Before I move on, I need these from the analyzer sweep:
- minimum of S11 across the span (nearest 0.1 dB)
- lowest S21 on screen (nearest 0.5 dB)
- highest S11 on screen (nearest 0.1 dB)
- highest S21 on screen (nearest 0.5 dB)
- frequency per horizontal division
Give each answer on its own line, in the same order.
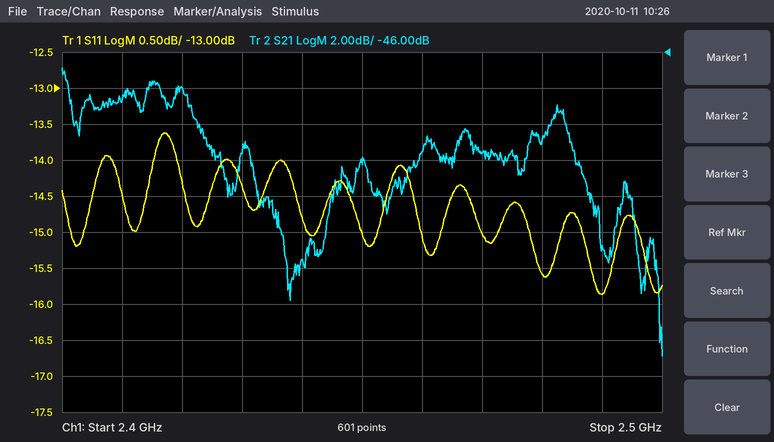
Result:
-15.9 dB
-63.0 dB
-13.6 dB
-47.0 dB
10 MHz
